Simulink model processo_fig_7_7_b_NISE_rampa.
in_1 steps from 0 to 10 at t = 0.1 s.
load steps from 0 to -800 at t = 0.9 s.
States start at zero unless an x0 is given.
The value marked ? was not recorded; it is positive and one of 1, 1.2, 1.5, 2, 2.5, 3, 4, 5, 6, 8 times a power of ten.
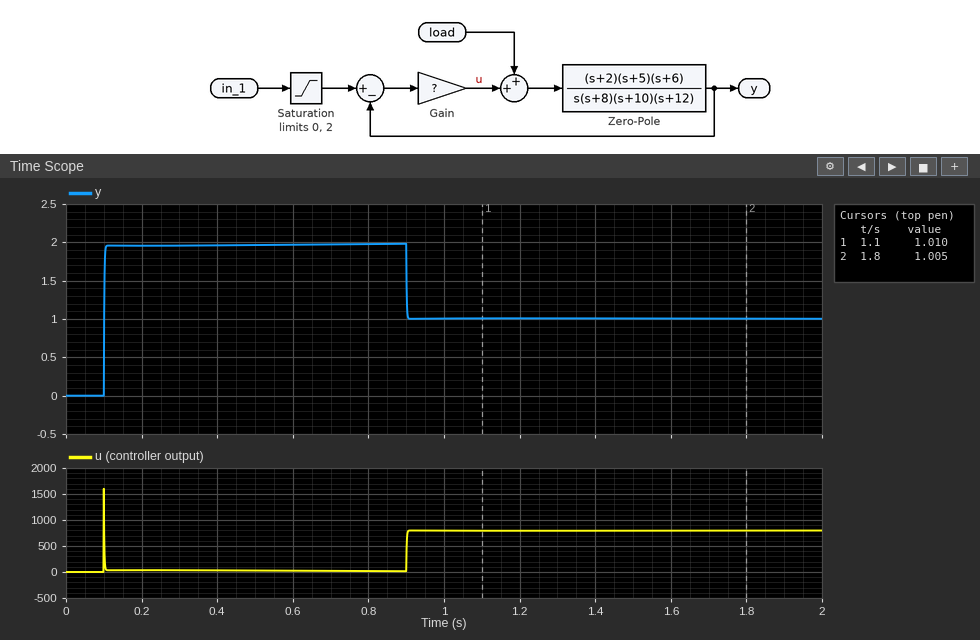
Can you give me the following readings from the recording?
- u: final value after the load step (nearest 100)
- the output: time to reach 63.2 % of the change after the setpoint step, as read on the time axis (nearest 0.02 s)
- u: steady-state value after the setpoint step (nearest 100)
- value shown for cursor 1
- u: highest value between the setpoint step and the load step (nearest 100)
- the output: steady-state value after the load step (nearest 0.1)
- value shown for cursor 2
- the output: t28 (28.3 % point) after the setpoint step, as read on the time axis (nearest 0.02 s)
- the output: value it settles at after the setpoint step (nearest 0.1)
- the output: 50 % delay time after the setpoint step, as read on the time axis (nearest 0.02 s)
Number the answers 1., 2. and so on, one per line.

1. 800
2. 0.10 s
3. 0
4. 1.010
5. 1600
6. 1.0
7. 1.005
8. 0.10 s
9. 2.0
10. 0.10 s
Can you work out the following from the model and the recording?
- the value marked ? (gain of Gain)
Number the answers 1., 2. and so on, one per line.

1. 800
